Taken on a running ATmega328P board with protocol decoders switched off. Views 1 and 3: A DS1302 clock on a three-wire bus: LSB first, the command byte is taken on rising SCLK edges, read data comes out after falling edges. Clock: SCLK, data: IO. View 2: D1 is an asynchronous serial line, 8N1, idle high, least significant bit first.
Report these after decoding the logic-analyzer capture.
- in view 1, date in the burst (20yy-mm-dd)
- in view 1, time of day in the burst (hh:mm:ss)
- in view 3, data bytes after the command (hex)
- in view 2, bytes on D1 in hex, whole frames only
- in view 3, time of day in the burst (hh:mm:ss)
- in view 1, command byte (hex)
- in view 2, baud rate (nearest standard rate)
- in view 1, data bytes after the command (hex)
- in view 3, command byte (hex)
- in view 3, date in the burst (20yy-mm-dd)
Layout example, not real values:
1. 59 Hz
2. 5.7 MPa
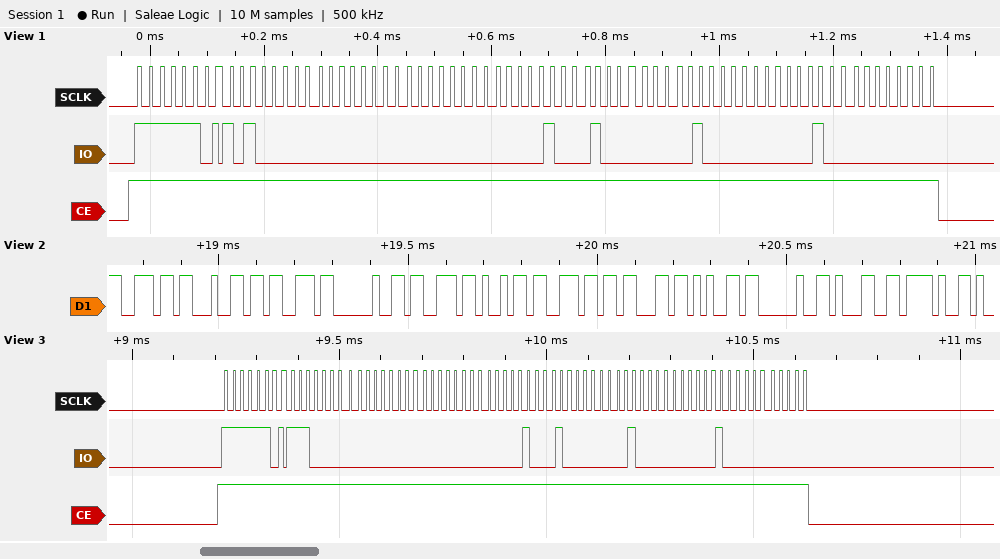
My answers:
1. 2020-02-20
2. 00:00:05
3. 07 00 00 20 02 04 20 00
4. 6E 64 73 20 73 69 6E 63 65 20 31 2F
5. 00:00:07
6. 0xBF
7. 57600 baud
8. 05 00 00 20 02 04 20 00
9. 0xBF
10. 2020-02-20
